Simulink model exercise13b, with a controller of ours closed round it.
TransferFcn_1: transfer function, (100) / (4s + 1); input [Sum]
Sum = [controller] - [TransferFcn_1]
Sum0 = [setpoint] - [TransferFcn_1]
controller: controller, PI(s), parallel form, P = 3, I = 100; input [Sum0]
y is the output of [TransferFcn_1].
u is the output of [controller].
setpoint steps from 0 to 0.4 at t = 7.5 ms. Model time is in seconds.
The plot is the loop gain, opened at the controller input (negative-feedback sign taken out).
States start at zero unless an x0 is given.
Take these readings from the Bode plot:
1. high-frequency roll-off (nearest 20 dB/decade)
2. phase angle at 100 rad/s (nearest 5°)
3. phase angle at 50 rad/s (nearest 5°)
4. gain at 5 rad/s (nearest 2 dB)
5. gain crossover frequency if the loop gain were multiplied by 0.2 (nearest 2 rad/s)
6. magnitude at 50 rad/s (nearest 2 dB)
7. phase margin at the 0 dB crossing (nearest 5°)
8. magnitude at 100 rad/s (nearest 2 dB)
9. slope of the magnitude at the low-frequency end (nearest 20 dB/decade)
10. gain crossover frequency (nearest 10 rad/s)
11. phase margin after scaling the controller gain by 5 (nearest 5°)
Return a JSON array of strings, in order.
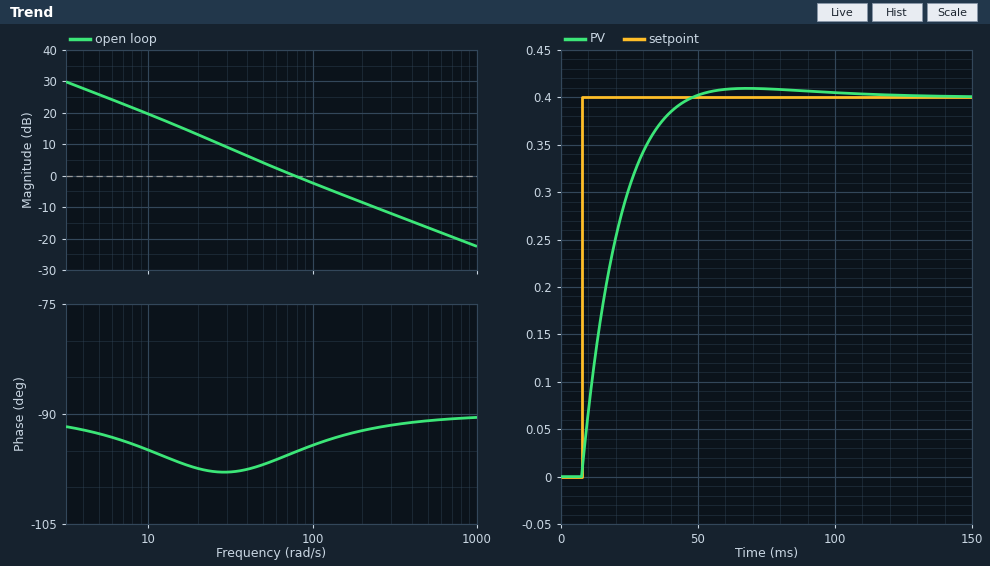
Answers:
["-20 dB/decade", "-95°", "-95°", "26 dB", "18 rad/s", "4 dB", "85°", "-2 dB", "-20 dB/decade", "80 rad/s", "90°"]
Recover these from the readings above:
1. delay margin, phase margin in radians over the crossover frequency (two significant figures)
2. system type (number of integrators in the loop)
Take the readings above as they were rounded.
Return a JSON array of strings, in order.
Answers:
["0.019 s", "1"]
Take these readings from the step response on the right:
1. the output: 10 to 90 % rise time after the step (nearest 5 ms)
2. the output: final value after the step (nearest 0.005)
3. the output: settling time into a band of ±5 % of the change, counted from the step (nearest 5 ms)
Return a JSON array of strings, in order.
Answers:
["25 ms", "0.400", "30 ms"]
